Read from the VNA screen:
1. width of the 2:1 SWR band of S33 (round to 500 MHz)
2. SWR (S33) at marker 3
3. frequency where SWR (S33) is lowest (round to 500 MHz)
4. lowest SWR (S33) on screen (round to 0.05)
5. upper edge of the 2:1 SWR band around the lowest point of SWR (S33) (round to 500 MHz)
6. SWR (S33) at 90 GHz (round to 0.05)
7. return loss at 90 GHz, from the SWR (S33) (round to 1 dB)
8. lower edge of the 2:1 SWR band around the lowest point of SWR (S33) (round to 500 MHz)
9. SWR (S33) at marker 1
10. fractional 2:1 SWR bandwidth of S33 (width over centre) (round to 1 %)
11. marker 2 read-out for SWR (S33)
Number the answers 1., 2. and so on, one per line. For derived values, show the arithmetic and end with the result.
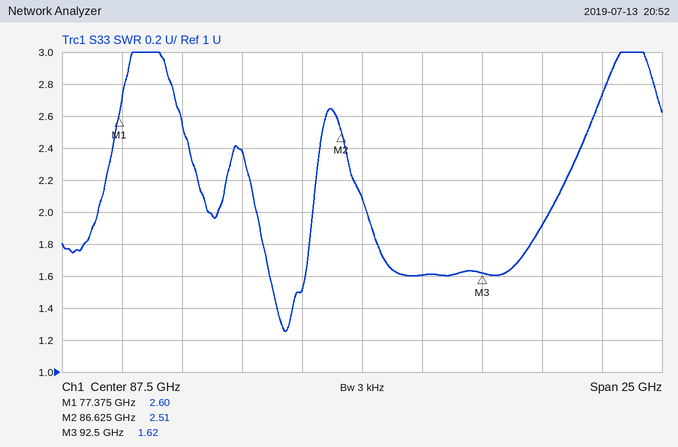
1. 85.5 GHz − 83.0 GHz = 2.5 GHz
2. 1.62
3. 84.5 GHz
4. 1.25
5. 85.5 GHz
6. 1.60
7. −20 log10((1.6 − 1)/(1.6 + 1)) ≈ 13 dB
8. 83.0 GHz
9. 2.60
10. 2.5 GHz / 84.25 GHz ≈ 3 %
11. 2.51
